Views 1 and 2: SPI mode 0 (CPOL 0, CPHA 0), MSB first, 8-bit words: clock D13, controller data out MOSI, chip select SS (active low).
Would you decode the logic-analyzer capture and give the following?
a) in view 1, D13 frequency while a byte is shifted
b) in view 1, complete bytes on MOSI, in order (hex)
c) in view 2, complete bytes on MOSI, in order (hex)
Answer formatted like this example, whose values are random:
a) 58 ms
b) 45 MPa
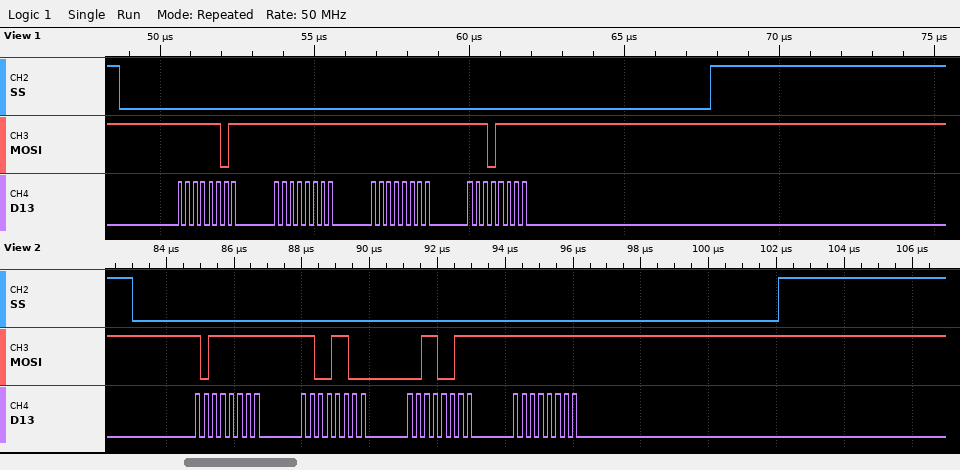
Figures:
a) 4 MHz
b) FD FF FF EF
c) BF CC 33 FF
